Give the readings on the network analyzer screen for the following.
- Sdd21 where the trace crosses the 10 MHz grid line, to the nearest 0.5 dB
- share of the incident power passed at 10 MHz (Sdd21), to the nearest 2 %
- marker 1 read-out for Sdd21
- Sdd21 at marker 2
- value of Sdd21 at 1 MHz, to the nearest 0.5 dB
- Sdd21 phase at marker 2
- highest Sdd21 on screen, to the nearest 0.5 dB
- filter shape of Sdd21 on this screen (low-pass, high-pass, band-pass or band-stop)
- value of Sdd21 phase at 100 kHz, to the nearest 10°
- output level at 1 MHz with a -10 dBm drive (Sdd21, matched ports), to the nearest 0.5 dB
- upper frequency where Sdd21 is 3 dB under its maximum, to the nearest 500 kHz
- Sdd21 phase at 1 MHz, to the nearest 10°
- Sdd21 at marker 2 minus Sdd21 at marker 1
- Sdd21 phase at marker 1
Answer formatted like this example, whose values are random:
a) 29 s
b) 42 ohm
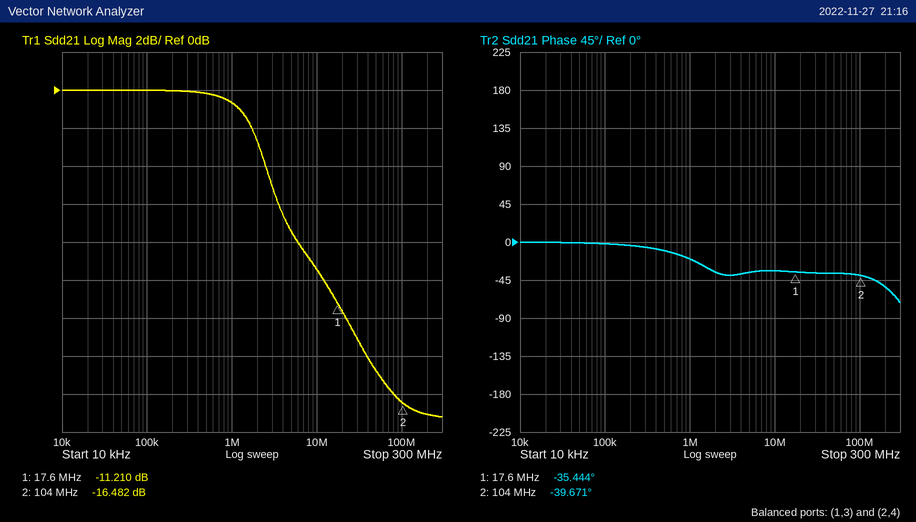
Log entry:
a) -9.5 dB
b) 12 %
c) -11.210 dB
d) -16.482 dB
e) -0.5 dB
f) -39.671°
g) 0.0 dB
h) low-pass
i) 0°
j) -10.5 dBm
k) 2.0 MHz
l) -20°
m) -5.272 dB
n) -35.444°
